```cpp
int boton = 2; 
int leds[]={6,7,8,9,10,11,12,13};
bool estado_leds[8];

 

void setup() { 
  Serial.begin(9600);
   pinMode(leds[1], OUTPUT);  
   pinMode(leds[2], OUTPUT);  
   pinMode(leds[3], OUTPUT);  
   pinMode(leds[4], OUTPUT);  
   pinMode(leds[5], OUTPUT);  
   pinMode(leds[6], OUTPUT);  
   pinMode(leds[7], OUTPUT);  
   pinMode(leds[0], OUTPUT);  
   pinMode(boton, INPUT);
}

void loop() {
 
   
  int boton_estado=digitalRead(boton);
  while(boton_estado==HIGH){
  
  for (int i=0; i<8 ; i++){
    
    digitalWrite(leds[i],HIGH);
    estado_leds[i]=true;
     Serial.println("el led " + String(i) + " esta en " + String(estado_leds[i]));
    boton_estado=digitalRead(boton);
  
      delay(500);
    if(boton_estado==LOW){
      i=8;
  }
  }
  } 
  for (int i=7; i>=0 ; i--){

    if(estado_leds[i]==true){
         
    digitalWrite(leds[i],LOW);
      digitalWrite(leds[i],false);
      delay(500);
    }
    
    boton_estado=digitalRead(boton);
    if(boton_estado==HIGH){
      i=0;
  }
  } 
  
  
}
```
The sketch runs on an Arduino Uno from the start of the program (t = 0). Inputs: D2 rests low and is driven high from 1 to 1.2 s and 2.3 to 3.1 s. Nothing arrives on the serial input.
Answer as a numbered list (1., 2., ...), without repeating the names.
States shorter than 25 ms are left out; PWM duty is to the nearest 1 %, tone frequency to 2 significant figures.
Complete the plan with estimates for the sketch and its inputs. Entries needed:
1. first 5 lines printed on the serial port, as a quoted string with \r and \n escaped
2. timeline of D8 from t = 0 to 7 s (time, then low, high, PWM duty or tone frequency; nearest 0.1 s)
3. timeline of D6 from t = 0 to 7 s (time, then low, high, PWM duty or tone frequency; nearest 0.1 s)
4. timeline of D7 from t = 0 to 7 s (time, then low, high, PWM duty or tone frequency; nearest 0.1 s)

1. "el led 0 esta en 1\r\nel led 1 esta en 1\r\nel led 0 esta en 1\r\nel led 1 esta en 1\r\nel led 2 esta en 1\r\n"
2. 0 s low; 3.5 s high; 4 s low
3. 0 s low; 1 s high; 5 s low
4. 0 s low; 1.5 s high; 2 s low; 3 s high; 4.5 s low
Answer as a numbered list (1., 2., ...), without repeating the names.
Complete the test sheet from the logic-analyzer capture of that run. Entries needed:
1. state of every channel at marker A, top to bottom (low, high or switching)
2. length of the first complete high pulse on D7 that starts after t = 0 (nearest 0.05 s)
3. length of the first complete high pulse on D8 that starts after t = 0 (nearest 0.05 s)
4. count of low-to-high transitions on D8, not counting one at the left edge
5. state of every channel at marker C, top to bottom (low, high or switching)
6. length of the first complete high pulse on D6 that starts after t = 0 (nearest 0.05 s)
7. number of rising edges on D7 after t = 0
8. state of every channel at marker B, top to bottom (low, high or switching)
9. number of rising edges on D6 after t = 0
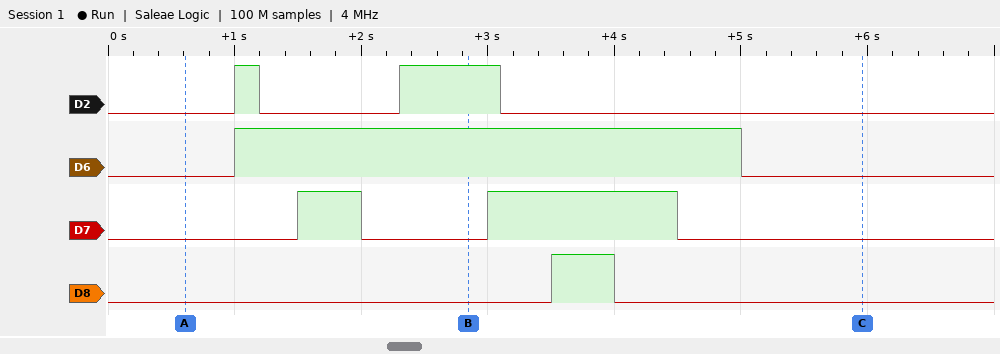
1. D2 low, D6 low, D7 low, D8 low
2. 0.50 s
3. 0.50 s
4. 1
5. D2 low, D6 low, D7 low, D8 low
6. 4.00 s
7. 2
8. D2 high, D6 high, D7 low, D8 low
9. 1
